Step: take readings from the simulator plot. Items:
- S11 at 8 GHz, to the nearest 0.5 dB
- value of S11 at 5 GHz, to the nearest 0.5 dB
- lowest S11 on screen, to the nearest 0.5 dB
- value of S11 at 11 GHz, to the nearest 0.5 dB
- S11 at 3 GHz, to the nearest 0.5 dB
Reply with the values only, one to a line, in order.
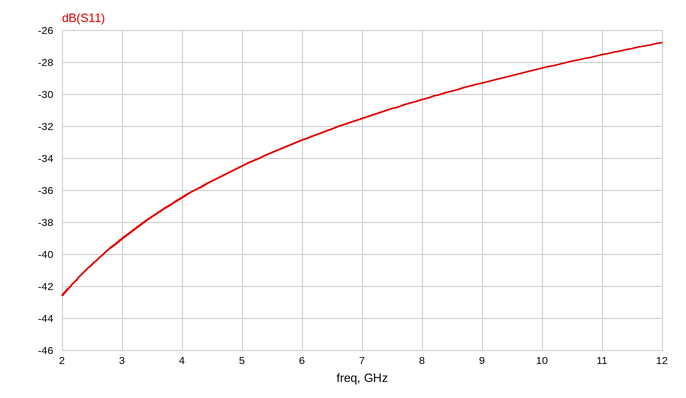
-30.5 dB
-34.5 dB
-42.5 dB
-27.5 dB
-39.0 dB
